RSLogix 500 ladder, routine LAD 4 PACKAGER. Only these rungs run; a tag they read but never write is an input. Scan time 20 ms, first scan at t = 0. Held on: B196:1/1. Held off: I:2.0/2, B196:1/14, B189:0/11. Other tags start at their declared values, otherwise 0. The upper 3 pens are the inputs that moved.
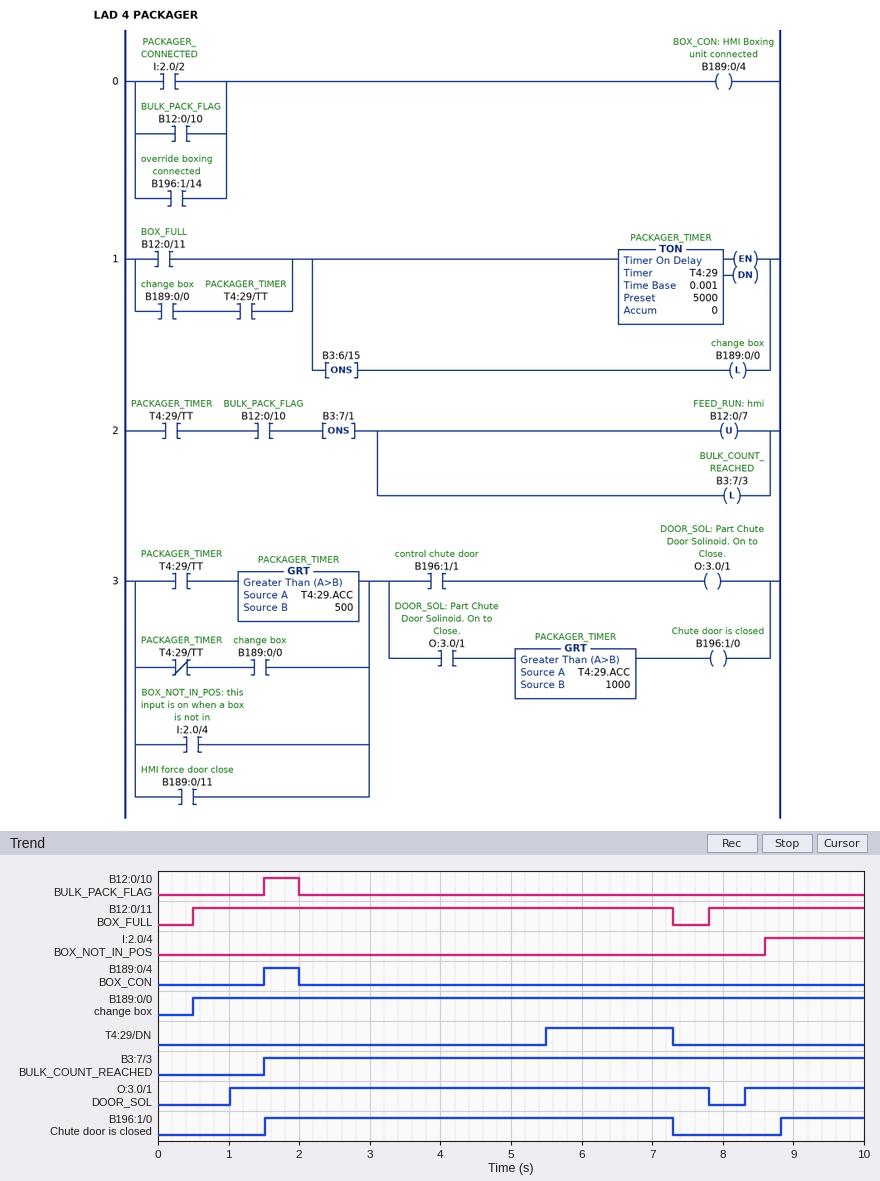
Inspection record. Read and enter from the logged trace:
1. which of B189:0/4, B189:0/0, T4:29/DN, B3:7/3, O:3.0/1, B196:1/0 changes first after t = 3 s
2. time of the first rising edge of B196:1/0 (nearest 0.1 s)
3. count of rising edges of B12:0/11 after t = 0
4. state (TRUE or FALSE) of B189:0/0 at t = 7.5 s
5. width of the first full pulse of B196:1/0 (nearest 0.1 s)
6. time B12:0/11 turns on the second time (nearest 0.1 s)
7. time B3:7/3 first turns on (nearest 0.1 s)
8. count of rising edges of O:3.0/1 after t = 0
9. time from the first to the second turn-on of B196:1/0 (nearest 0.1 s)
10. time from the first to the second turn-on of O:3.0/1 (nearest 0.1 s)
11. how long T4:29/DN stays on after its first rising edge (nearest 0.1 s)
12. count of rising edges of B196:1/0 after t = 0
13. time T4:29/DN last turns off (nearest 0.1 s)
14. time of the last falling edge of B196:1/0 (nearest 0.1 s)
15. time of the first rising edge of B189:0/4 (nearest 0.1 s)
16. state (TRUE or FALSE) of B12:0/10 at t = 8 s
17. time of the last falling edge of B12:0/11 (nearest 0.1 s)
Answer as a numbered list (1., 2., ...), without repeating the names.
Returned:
1. T4:29/DN
2. 1.5 s
3. 2
4. TRUE
5. 5.8 s
6. 7.8 s
7. 1.5 s
8. 2
9. 7.3 s
10. 7.3 s
11. 1.8 s
12. 2
13. 7.3 s
14. 7.3 s
15. 1.5 s
16. FALSE
17. 7.3 s
